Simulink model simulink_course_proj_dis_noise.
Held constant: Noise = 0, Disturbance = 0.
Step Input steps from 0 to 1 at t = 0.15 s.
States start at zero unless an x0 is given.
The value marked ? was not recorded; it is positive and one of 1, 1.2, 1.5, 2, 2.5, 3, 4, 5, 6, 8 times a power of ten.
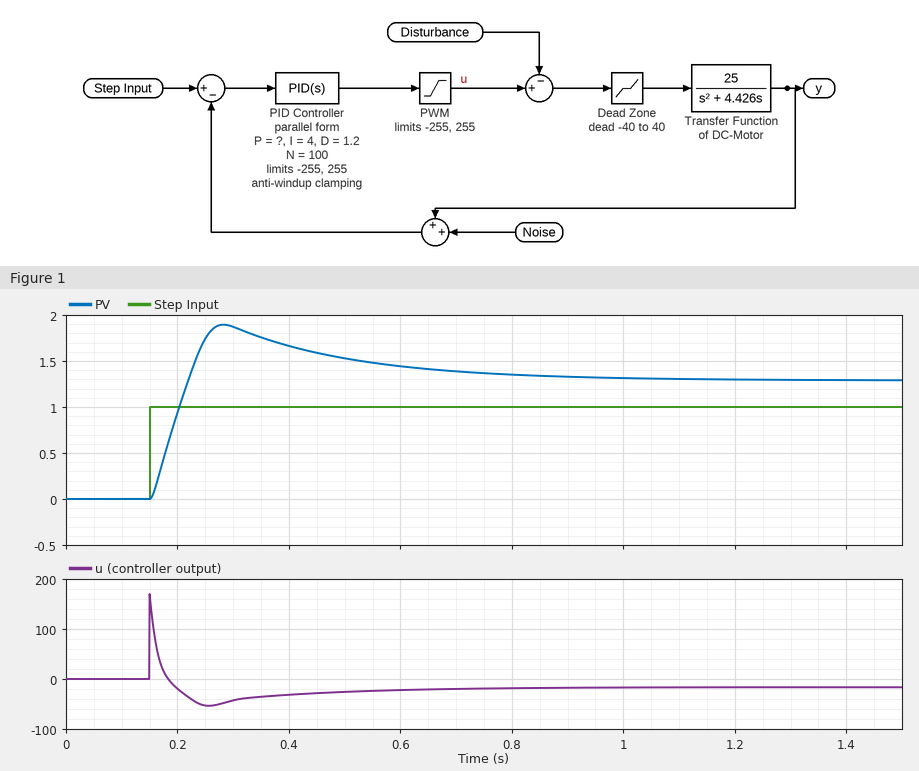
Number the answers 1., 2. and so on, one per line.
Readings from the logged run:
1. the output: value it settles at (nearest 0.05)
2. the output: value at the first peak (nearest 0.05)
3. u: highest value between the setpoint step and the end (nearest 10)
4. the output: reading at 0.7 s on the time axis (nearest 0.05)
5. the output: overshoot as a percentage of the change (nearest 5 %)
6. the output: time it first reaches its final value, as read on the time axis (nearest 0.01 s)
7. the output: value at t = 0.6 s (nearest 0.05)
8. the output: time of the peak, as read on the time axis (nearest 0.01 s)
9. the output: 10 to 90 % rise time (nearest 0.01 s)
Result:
1. 1.30
2. 1.90
3. 170
4. 1.40
5. 45 %
6. 0.22 s
7. 1.45
8. 0.28 s
9. 0.05 s
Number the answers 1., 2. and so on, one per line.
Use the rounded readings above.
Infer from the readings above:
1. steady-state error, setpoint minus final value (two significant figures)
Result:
1. -0.30
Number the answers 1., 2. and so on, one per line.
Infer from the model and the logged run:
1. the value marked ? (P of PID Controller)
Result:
1. 50
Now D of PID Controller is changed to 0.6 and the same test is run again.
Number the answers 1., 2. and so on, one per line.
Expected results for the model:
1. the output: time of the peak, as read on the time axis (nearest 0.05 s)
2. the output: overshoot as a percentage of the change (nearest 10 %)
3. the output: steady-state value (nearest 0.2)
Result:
1. 0.35 s
2. 70 %
3. 1.2
